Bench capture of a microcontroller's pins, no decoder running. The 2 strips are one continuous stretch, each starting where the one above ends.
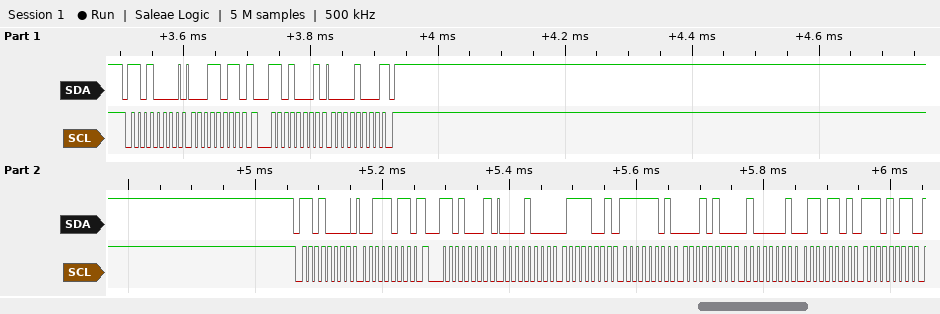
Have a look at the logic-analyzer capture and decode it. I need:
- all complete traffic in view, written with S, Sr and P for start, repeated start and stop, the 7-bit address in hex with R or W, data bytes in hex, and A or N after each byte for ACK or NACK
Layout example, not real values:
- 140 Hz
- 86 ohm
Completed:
- S 68W A 1B A Sr 68R A 08 N P S 68W A 3B A Sr 68R A 08 A 79 A FD A 14 A 41 A 6D A EB A
